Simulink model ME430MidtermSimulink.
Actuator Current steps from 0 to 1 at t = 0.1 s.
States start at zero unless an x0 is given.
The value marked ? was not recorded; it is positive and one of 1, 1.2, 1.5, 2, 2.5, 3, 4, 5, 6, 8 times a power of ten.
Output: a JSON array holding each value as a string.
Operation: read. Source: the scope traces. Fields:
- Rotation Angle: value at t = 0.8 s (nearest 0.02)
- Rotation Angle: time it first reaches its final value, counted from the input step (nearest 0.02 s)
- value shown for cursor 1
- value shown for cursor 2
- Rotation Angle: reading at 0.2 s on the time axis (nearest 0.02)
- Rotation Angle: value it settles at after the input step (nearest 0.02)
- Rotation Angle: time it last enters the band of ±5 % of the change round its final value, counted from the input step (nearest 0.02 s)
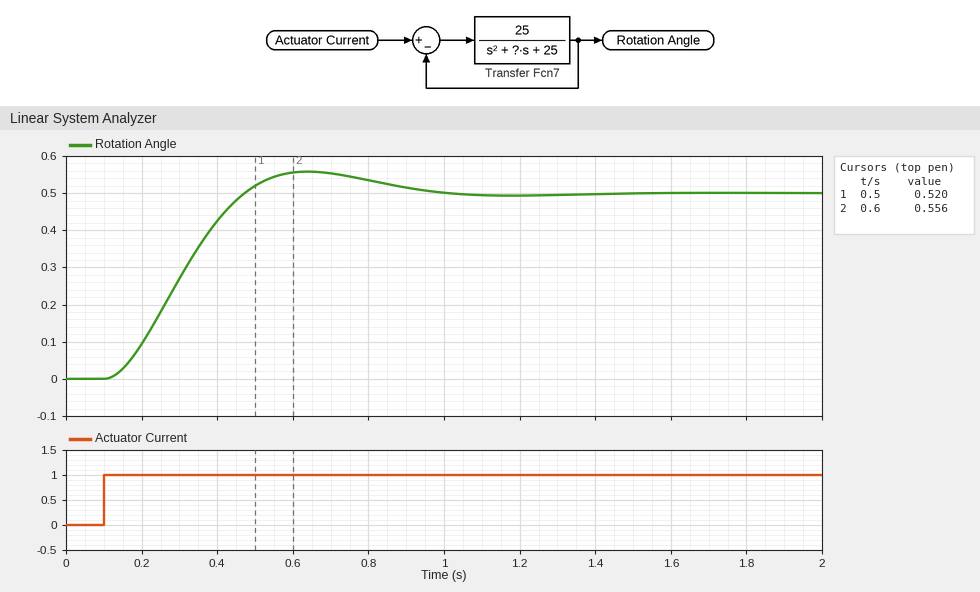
["0.54", "0.38 s", "0.520", "0.556", "0.10", "0.50", "0.74 s"]
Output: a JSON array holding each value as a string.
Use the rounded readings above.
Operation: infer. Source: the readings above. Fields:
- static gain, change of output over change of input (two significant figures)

["0.50"]
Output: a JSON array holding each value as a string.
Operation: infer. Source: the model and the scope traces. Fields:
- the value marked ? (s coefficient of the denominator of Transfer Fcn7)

["8"]
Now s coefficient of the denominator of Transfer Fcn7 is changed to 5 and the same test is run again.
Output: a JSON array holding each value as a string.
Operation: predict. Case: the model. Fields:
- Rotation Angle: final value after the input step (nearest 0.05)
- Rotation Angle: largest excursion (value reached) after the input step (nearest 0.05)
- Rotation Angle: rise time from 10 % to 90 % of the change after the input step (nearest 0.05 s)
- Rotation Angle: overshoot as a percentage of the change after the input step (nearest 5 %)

["0.50", "0.65", "0.20 s", "30 %"]
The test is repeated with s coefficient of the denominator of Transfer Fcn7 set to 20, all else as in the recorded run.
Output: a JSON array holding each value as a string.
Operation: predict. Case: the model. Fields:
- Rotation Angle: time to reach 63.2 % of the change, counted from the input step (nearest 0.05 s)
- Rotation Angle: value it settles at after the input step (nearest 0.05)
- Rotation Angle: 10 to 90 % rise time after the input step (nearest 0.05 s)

["0.40 s", "0.50", "0.75 s"]
